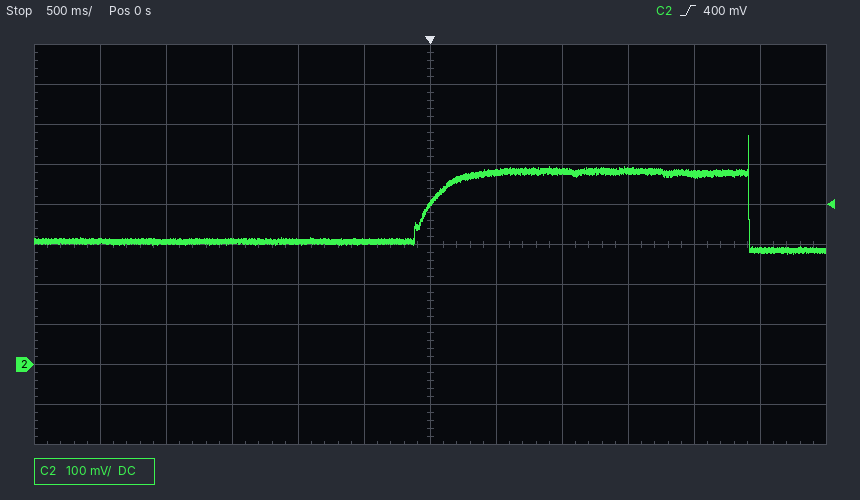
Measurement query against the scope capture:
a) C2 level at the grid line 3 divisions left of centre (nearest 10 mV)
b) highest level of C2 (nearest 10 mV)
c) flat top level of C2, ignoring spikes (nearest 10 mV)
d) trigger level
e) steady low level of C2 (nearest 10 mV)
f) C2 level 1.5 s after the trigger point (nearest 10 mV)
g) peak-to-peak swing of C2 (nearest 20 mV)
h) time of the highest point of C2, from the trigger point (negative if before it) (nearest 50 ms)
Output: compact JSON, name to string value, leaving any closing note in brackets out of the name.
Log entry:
{"C2 level at the grid line 3 divisions left of centre": "310 mV", "highest level of C2": "570 mV", "flat top level of C2, ignoring spikes": "480 mV", "trigger level": "400 mV", "steady low level of C2": "310 mV", "C2 level 1.5 s after the trigger point": "480 mV", "peak-to-peak swing of C2": "300 mV", "time of the highest point of C2, from the trigger point (negative if before it)": "+2.40 s"}
